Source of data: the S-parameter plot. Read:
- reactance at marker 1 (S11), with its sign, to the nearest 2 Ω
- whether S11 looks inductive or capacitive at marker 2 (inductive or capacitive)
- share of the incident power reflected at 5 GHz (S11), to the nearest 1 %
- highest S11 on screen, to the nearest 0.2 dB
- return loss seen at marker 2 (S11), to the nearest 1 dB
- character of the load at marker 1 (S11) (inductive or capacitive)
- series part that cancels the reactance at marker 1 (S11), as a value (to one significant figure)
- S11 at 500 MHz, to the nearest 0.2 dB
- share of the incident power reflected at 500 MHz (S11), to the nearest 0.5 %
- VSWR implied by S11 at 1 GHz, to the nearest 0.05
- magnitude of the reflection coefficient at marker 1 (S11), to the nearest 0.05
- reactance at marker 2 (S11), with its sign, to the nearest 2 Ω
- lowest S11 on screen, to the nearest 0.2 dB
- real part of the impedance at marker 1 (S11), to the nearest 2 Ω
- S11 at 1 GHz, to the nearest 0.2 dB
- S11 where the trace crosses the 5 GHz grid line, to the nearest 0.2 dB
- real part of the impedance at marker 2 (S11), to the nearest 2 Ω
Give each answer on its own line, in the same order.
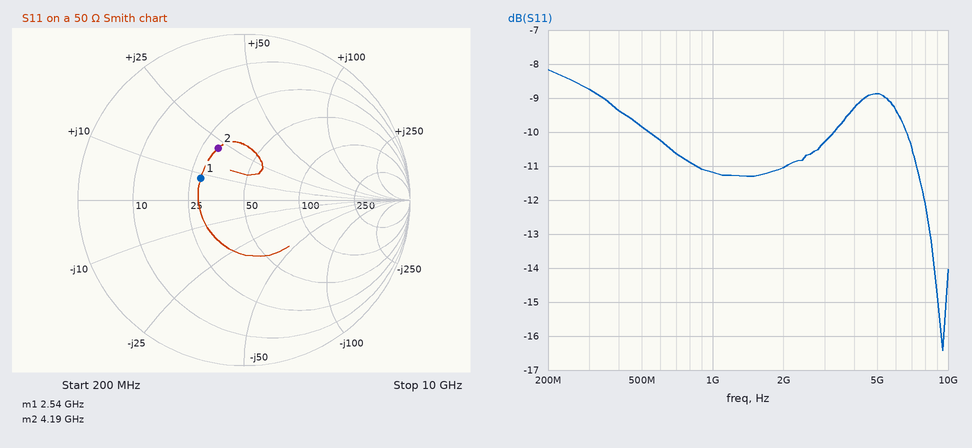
+8 Ω
inductive
13 %
-8.2 dB
9 dB
inductive
8 pF
-9.8 dB
10.5 %
1.75
0.30
+22 Ω
-16.4 dB
28 Ω
-11.2 dB
-8.8 dB
30 Ω
